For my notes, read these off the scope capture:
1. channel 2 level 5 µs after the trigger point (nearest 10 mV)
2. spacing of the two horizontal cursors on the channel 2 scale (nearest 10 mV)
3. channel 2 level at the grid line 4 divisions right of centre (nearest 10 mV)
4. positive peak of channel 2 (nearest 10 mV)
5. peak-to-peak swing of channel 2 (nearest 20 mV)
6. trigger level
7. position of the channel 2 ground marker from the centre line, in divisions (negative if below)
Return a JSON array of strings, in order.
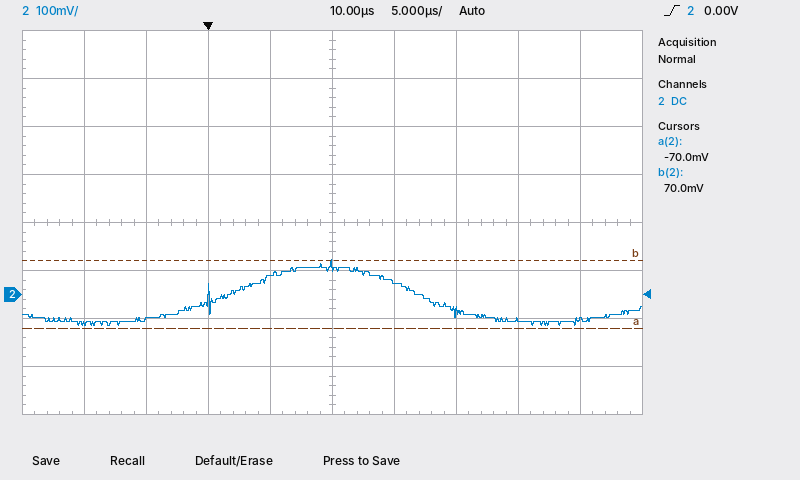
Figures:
["40 mV", "140 mV", "-50 mV", "70 mV", "140 mV", "0.00 V", "-1.5 div"]
